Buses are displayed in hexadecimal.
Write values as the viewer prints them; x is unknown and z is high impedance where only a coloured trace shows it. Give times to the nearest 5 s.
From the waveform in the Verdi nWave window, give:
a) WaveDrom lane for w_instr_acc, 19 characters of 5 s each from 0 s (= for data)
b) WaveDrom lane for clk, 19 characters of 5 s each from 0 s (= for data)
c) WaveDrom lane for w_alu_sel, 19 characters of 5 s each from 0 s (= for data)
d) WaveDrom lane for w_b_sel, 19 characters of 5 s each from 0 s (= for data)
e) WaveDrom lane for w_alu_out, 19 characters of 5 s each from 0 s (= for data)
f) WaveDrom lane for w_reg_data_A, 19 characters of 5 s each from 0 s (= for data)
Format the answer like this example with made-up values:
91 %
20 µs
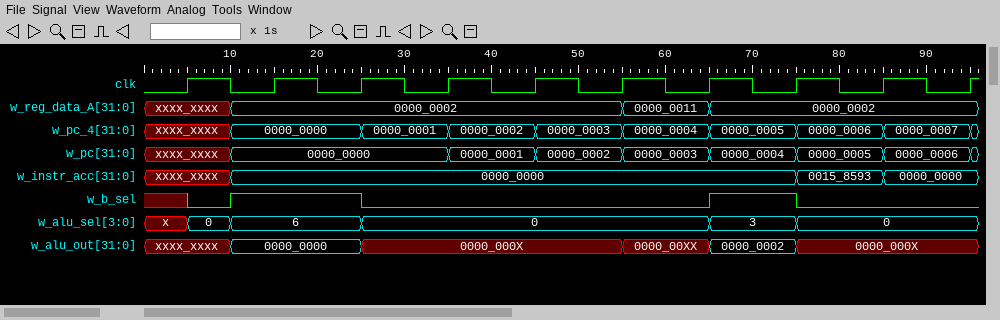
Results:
{name: 'w_instr_acc', wave: 'x.=............=.=.', data: '0000_0000 0015_8593 0000_0000'}
{name: 'clk', wave: '0101010101010101010'}
{name: 'w_alu_sel', wave: 'x==..=.......=.=...', data: '0 6 0 3 0'}
{name: 'w_b_sel', wave: 'x01..0.......1.0...'}
{name: 'w_alu_out', wave: 'x.=..=.....=.=.=...', data: '0000_0000 0000_000X 0000_00XX 0000_0002 0000_000X'}
{name: 'w_reg_data_A', wave: 'x.=........=.=.....', data: '0000_0002 0000_0011 0000_0002'}
